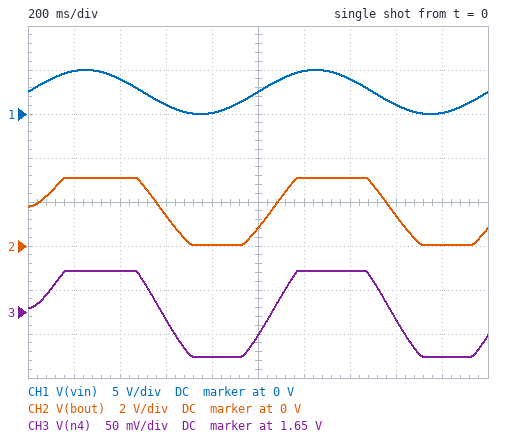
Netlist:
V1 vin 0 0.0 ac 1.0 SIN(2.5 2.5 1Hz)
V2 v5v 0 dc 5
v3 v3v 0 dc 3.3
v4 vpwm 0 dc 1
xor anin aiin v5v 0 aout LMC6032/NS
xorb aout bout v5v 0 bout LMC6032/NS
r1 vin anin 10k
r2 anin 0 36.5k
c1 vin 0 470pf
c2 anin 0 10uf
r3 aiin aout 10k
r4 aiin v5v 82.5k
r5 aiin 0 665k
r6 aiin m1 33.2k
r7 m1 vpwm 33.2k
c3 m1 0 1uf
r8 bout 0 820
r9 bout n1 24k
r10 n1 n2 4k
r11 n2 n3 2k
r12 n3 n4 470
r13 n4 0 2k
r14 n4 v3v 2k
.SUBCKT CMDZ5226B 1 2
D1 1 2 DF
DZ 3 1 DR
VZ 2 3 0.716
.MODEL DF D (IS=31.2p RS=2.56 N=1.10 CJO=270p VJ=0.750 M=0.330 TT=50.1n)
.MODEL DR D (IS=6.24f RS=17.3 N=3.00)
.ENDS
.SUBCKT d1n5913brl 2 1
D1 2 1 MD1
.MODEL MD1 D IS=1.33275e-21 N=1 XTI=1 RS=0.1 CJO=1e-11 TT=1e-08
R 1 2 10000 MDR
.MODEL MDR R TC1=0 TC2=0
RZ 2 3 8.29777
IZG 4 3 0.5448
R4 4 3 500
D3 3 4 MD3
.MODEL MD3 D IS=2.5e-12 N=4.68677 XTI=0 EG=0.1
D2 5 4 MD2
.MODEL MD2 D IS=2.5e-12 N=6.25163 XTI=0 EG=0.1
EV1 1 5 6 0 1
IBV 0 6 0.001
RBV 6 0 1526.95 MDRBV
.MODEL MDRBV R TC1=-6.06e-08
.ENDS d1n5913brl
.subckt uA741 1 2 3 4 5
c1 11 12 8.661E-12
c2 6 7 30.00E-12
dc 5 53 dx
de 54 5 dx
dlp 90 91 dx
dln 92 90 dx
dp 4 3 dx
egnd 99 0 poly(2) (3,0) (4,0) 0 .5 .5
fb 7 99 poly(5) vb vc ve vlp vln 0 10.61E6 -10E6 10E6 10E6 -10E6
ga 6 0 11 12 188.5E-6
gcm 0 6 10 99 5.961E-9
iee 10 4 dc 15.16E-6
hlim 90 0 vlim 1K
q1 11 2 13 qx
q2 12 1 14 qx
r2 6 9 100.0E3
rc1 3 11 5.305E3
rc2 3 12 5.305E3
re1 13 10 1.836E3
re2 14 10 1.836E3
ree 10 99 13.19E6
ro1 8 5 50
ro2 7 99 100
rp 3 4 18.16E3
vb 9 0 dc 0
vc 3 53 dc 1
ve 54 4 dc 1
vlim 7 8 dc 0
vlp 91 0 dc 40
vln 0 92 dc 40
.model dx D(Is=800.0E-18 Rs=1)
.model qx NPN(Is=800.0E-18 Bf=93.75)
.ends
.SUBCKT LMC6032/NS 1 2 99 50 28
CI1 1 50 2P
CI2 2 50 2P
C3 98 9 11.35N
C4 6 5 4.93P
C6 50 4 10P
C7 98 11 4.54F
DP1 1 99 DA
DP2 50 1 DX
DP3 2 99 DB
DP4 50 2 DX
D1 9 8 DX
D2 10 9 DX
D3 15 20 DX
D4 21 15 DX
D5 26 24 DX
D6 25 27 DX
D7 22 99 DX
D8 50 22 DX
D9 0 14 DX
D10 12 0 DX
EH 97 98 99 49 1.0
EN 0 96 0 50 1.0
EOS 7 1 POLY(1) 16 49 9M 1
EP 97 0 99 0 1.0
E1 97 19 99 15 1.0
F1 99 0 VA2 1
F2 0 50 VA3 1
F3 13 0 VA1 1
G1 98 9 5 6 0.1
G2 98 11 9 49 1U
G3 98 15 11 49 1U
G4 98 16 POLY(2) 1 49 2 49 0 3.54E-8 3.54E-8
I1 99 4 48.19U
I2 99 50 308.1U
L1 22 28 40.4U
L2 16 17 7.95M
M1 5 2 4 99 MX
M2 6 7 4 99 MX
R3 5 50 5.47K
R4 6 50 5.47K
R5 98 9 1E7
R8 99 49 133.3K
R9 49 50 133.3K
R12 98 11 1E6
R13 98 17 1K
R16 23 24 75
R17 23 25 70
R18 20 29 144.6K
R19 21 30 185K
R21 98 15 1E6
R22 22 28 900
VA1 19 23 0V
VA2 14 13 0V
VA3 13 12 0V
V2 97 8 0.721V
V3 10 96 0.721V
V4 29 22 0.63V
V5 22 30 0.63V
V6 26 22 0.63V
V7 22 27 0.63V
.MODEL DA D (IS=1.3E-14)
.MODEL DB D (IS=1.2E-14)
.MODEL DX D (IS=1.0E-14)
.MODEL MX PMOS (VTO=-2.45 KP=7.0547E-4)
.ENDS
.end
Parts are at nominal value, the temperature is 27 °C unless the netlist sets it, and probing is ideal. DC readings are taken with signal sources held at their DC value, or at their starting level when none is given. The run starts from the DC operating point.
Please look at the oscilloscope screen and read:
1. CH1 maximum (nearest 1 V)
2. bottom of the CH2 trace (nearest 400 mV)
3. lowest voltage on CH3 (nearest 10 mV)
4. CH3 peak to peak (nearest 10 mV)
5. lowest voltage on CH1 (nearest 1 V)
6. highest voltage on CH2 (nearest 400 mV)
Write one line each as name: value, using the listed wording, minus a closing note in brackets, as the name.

CH1 maximum: 5 V
bottom of the CH2 trace: 0 V
lowest voltage on CH3: 1.60 V
CH3 peak to peak: 100 mV
lowest voltage on CH1: 0 V
highest voltage on CH2: 3.2 V
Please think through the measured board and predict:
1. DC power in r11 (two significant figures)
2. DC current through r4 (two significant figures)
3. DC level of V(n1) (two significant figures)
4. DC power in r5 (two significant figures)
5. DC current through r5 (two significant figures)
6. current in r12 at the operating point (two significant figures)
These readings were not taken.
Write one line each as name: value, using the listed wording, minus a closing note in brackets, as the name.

DC power in r11: 5.3 µW
DC current through r4: 54 µA
DC level of V(n1): 1.3 V
DC power in r5: 500 nW
DC current through r5: 870 nA
current in r12 at the operating point: 51 µA
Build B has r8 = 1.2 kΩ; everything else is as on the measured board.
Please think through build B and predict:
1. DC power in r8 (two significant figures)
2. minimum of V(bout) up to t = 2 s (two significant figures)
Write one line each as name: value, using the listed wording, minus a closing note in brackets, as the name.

DC power in r8: 970 nW
minimum of V(bout) up to t = 2 s: 34 mV
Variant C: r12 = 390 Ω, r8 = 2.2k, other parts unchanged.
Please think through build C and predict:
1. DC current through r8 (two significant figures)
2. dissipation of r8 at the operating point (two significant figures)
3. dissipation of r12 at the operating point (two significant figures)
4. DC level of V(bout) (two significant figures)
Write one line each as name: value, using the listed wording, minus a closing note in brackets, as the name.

DC current through r8: 16 µA
dissipation of r8 at the operating point: 550 nW
dissipation of r12 at the operating point: 1.0 µW
DC level of V(bout): 35 mV
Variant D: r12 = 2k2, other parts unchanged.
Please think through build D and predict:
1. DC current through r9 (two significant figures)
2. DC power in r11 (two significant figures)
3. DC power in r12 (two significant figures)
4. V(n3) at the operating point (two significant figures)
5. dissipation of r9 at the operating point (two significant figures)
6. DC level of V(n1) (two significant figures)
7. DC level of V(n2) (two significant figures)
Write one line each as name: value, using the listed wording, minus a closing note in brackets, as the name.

DC current through r9: 49 µA
DC power in r11: 4.7 µW
DC power in r12: 5.2 µW
V(n3) at the operating point: 1.5 V
dissipation of r9 at the operating point: 57 µW
DC level of V(n1): 1.2 V
DC level of V(n2): 1.4 V
